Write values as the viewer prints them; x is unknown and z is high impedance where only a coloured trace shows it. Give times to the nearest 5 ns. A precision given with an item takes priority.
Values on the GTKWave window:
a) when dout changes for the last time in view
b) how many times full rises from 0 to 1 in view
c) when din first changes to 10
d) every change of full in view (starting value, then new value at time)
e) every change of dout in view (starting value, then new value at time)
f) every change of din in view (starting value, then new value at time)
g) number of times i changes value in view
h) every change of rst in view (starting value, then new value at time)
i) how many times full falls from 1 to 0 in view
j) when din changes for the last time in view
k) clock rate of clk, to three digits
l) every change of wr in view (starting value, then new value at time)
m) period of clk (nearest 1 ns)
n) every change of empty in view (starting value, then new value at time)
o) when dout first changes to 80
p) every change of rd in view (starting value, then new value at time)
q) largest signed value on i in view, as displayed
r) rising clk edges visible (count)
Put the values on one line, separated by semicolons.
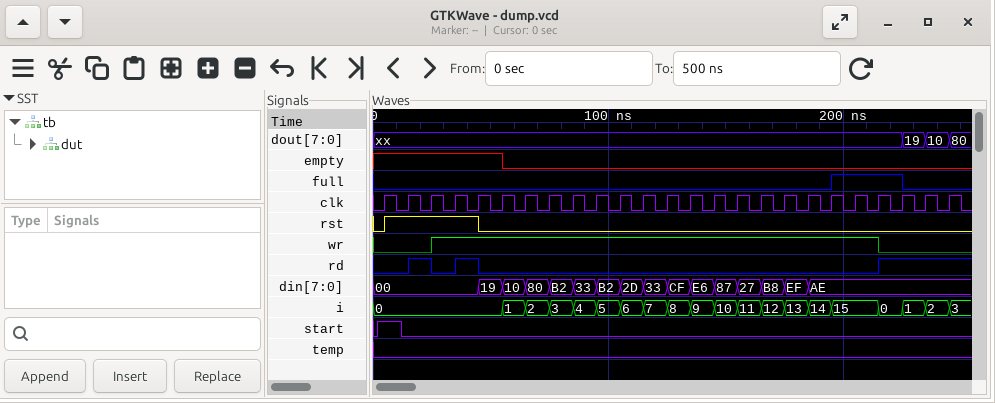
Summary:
245 ns; 1; 55 ns; 0, 1 at 195 ns, 0 at 225 ns; xx, 19 at 225 ns, 10 at 235 ns, 80 at 245 ns; 00, 19 at 45 ns, 10 at 55 ns, 80 at 65 ns, B2 at 75 ns, 33 at 85 ns, B2 at 95 ns, 2D at 105 ns, 33 at 115 ns, CF at 125 ns, E6 at 135 ns, 87 at 145 ns, 27 at 155 ns, B8 at 165 ns, EF at 175 ns, AE at 185 ns; 19; 0, 1 at 5 ns, 0 at 45 ns; 1; 185 ns; 100 MHz; 0, 1 at 25 ns, 0 at 215 ns; 10 ns; 1, 0 at 55 ns; 245 ns; 0, 1 at 15 ns, 0 at 25 ns, 1 at 35 ns, 0 at 45 ns, 1 at 215 ns; 15; 25
